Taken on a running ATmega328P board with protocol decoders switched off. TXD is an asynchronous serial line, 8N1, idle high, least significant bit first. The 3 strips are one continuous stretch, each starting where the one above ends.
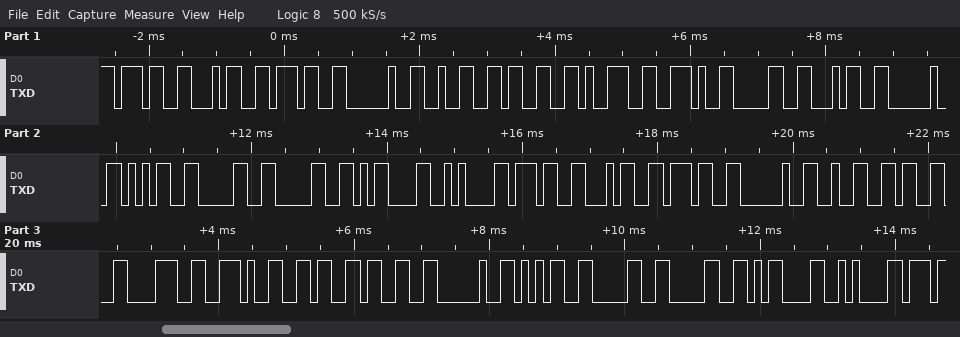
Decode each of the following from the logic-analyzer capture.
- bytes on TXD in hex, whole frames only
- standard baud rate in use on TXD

37 34 37 20 32 33 39 2E 30 34 20 35 30 30 0D 0A 37 34 37 20 32 33 38 2E 36 33 20 35 30 30 0D 0A
9600 baud
